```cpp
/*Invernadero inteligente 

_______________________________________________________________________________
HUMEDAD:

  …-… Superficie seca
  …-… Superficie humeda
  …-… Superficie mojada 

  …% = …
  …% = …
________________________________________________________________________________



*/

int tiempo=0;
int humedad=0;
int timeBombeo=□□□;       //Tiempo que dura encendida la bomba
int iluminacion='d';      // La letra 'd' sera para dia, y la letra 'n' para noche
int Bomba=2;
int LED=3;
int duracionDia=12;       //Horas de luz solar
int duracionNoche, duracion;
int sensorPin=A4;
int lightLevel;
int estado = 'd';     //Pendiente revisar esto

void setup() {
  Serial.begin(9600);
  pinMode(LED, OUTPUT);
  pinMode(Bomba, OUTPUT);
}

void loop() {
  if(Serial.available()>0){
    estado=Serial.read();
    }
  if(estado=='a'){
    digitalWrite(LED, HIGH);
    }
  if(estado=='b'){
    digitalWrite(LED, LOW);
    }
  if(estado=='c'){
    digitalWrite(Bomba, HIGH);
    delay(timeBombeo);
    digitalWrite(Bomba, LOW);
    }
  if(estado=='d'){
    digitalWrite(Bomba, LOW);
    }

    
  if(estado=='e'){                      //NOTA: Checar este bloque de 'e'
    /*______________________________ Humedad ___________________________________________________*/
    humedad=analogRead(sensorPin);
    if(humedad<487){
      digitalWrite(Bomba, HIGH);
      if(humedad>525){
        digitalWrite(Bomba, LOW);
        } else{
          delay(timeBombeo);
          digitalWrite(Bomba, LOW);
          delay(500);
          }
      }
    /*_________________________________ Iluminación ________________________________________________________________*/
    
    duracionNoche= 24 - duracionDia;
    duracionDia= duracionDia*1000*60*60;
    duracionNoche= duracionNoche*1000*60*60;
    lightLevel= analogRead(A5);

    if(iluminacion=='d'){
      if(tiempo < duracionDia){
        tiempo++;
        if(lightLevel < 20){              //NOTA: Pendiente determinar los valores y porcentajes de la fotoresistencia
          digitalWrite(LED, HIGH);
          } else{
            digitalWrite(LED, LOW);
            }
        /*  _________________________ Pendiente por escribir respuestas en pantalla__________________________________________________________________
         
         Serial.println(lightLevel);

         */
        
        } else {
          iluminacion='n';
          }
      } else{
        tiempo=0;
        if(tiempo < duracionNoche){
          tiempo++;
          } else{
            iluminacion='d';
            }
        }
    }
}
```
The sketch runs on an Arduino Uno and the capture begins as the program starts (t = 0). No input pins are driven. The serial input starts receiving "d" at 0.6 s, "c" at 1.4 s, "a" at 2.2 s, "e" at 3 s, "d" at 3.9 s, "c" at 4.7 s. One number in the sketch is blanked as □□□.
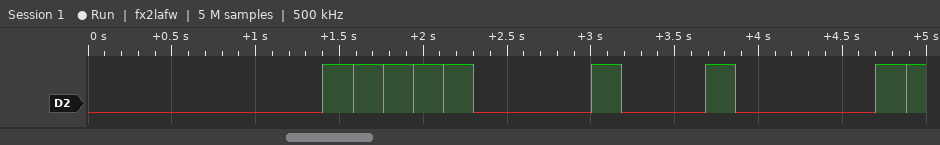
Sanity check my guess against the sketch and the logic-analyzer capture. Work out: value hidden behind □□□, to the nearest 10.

180
